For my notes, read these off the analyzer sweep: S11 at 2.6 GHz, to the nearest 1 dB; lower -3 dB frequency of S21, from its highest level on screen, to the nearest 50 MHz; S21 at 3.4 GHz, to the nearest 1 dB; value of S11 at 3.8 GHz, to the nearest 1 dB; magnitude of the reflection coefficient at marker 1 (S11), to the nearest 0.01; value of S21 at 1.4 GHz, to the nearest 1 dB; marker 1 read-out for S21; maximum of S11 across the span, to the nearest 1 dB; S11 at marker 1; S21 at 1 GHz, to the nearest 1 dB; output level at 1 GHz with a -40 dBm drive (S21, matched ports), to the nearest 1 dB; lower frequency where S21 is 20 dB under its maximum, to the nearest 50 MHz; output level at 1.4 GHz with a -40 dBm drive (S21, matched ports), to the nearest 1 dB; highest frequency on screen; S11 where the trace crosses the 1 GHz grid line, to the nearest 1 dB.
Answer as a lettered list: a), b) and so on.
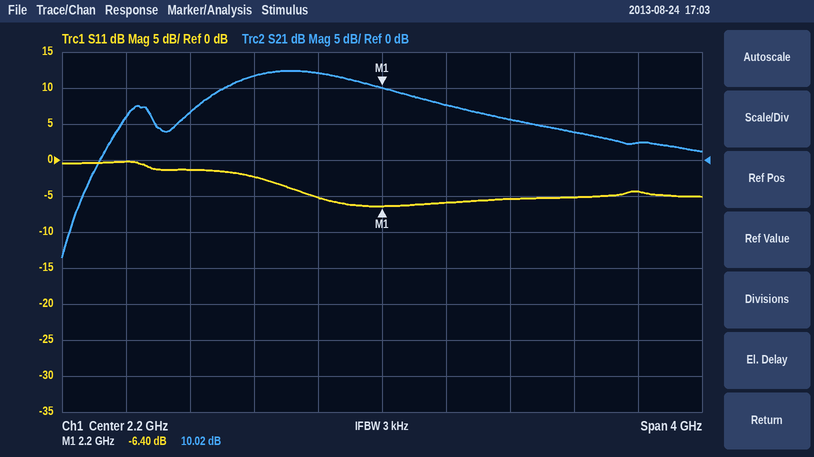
a) -6 dB
b) 1.15 GHz
c) 4 dB
d) -4 dB
e) 0.48
f) 12 dB
g) 10.02 dB
h) 0 dB
i) -6.40 dB
j) 7 dB
k) -33 dBm
l) 300 MHz
m) -28 dBm
n) 4.2 GHz
o) -1 dB
